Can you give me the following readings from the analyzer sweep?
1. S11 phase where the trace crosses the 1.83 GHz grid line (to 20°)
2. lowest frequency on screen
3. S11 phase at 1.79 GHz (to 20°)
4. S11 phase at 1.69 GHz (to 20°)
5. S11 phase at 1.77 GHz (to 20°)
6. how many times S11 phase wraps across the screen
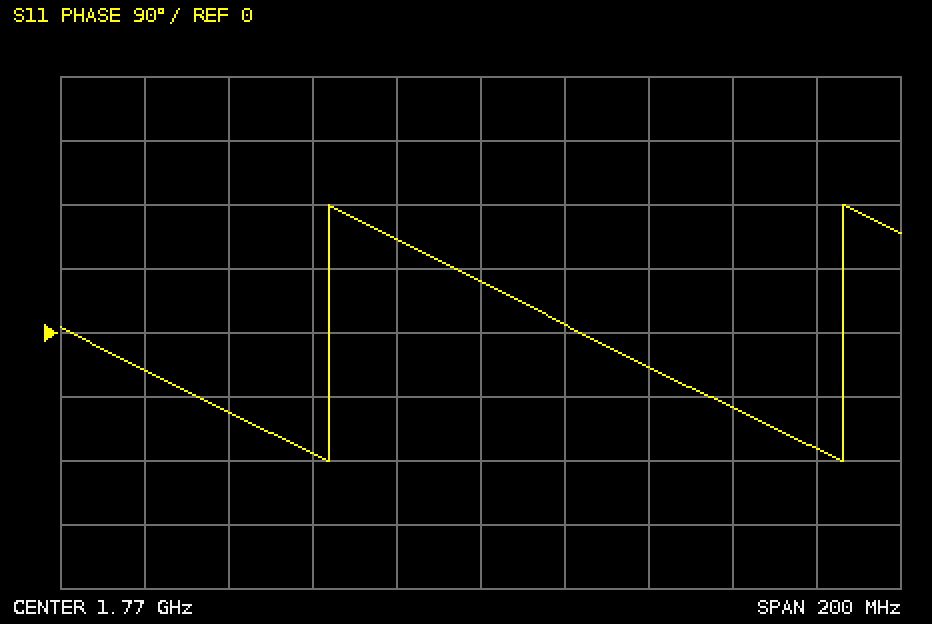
-100°
1.67 GHz
20°
-60°
80°
2
